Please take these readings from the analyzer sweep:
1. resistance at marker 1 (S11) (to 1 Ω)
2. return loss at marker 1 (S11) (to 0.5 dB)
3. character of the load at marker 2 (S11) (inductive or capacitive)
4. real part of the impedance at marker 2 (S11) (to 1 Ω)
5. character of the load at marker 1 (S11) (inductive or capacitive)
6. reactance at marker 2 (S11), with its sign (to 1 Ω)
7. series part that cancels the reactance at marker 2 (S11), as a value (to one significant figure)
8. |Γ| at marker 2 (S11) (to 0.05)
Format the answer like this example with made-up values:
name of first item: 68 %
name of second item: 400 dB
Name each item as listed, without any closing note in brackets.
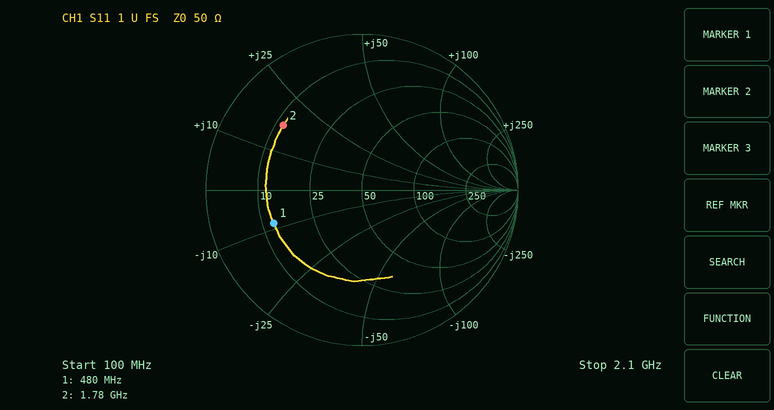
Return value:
resistance at marker 1 (S11): 13 Ω
return loss at marker 1 (S11): 4.5 dB
character of the load at marker 2 (S11): inductive
real part of the impedance at marker 2 (S11): 12 Ω
character of the load at marker 1 (S11): capacitive
reactance at marker 2 (S11), with its sign: +17 Ω
series part that cancels the reactance at marker 2 (S11), as a value: 5 pF
|Γ| at marker 2 (S11): 0.65
